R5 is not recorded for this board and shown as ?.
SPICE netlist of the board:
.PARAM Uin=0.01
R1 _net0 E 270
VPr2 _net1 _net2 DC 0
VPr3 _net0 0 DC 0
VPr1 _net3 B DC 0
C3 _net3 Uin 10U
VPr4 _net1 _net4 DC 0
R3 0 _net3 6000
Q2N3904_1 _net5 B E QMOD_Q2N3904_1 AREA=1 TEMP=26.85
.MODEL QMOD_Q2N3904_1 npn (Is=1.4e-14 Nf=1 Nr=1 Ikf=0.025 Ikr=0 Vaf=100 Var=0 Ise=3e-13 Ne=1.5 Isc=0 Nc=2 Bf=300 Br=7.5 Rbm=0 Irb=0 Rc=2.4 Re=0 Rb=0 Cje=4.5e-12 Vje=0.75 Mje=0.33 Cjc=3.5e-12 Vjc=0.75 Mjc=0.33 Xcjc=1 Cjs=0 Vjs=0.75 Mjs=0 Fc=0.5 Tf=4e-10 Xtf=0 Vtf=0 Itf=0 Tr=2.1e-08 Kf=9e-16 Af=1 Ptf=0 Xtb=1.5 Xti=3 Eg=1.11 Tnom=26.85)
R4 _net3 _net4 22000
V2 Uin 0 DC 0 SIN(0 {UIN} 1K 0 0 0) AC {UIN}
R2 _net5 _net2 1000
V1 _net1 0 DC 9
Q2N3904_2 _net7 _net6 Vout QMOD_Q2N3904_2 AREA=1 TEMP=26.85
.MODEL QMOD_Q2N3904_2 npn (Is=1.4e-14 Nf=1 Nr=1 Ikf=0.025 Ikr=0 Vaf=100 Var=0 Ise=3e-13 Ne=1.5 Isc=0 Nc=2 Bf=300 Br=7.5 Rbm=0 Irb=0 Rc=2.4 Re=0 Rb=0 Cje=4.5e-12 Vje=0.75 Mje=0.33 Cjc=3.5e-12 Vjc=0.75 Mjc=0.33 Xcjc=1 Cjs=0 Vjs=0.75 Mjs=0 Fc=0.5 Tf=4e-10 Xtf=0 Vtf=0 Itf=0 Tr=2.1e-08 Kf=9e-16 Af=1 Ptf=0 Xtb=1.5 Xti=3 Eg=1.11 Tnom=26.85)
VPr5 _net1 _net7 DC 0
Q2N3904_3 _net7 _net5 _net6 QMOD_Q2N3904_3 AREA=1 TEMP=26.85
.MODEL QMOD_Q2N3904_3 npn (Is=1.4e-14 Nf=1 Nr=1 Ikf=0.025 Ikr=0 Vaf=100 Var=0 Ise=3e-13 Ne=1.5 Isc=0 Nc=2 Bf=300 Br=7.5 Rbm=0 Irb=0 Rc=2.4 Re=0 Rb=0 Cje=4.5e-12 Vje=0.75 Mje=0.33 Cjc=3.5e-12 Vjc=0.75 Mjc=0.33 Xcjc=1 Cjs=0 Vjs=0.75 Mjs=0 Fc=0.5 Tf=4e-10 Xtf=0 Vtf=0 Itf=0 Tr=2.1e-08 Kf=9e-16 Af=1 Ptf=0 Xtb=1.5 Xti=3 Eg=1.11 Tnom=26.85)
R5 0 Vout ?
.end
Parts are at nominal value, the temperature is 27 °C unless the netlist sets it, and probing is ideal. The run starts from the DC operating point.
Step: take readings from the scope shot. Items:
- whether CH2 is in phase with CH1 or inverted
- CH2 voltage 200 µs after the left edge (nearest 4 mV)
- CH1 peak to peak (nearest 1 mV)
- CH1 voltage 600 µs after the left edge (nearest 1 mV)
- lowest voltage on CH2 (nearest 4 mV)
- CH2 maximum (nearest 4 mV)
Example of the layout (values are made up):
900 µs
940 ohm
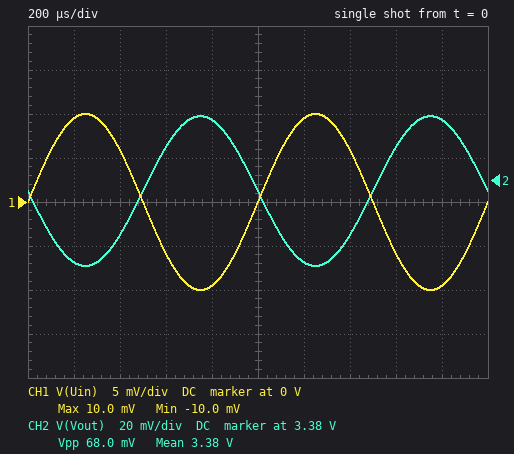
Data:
inverted
3.344 V
20 mV
-6 mV
3.340 V
3.408 V
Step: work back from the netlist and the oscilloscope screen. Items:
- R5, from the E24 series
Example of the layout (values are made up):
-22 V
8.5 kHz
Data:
18 Ω
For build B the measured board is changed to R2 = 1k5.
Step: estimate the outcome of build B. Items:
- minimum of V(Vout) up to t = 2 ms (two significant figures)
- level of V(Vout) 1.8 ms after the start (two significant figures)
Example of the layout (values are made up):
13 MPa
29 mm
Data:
1.4 V
1.5 V
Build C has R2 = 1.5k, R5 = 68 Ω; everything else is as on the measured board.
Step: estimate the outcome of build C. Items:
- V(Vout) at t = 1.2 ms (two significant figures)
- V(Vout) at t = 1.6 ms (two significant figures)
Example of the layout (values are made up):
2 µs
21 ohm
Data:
1.5 V
1.6 V
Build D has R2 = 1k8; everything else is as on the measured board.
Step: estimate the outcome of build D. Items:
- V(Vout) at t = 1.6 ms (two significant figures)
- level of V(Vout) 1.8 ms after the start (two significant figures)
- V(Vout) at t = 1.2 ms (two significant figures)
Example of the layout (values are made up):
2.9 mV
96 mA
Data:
410 mV
430 mV
330 mV
